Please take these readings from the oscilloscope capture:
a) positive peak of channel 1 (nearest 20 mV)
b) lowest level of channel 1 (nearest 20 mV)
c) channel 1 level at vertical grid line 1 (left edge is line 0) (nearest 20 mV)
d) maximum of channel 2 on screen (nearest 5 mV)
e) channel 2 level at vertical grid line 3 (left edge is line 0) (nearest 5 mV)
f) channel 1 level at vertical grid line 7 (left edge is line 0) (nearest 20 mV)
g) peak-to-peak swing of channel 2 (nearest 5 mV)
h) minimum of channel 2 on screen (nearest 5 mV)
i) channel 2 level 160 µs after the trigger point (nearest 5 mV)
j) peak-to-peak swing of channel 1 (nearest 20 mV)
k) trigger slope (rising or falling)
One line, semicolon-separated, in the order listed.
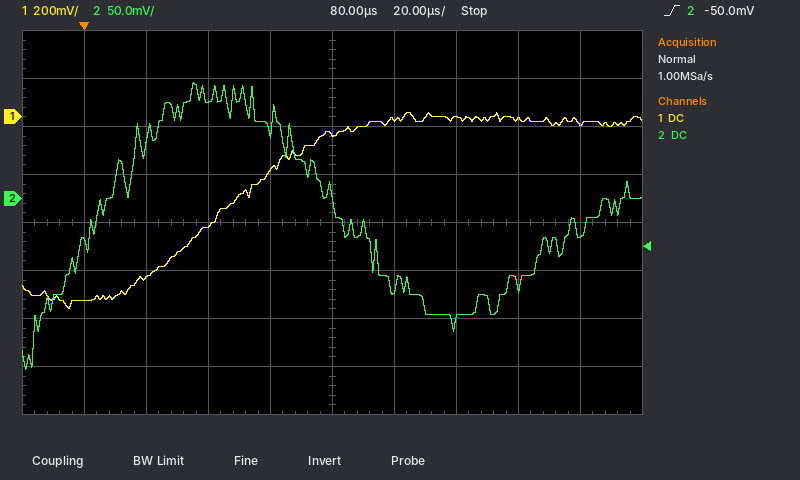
20 mV; -800 mV; -760 mV; 120 mV; 100 mV; 0 mV; 300 mV; -180 mV; -40 mV; 820 mV; rising
